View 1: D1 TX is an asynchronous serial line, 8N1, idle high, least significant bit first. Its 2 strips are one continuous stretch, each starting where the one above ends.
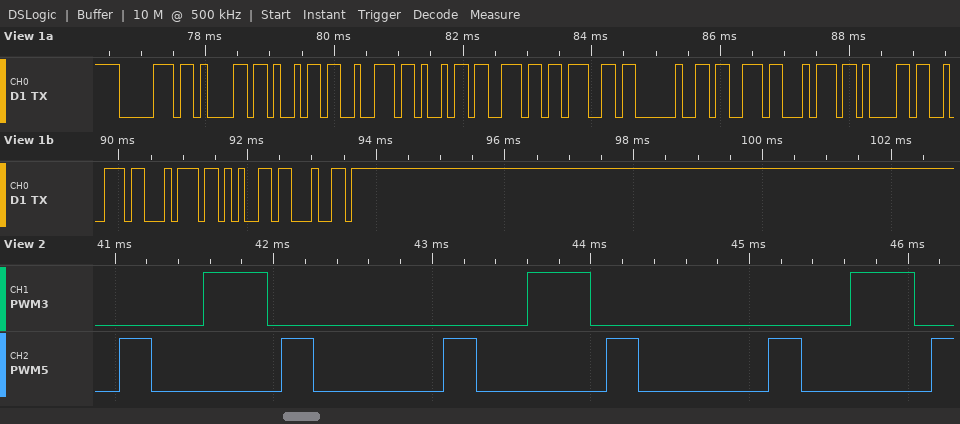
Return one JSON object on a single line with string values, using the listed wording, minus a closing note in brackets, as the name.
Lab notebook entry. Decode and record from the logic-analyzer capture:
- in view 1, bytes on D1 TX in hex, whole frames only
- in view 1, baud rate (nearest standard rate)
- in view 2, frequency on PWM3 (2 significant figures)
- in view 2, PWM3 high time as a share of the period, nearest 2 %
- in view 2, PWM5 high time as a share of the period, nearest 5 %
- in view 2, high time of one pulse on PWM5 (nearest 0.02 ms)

{"in view 1, bytes on D1 TX in hex, whole frames only": "0x70 0x61 0x69 0x72 0x69 0x6E 0x67 0x20 0x73 0x74 0x61 0x72 0x74 0x65 0x64", "in view 1, baud rate": "9600 baud", "in view 2, frequency on PWM3": "490 Hz", "in view 2, PWM3 high time as a share of the period, nearest 2 %": "20 %", "in view 2, PWM5 high time as a share of the period, nearest 5 %": "20 %", "in view 2, high time of one pulse on PWM5": "0.20 ms"}
